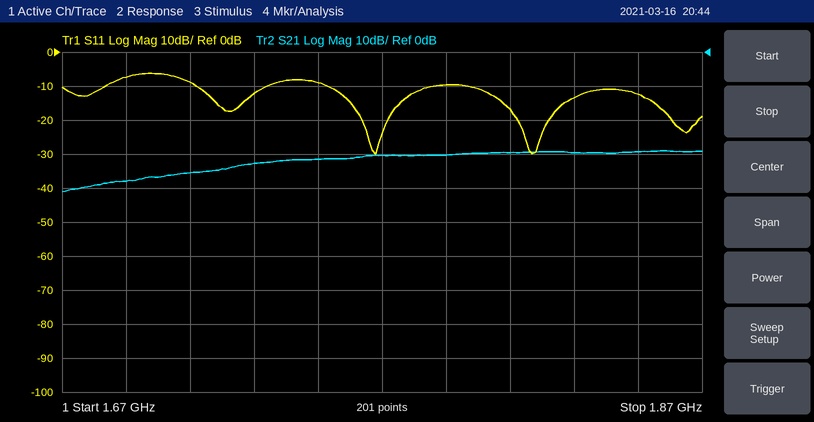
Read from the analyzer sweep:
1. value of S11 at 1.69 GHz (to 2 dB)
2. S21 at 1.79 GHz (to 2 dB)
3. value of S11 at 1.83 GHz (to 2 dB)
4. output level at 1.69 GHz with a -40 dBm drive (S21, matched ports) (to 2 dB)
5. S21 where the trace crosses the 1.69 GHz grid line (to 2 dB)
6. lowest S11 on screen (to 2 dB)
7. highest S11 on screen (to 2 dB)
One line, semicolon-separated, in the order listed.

-8 dB; -30 dB; -14 dB; -78 dBm; -38 dB; -30 dB; -6 dB
